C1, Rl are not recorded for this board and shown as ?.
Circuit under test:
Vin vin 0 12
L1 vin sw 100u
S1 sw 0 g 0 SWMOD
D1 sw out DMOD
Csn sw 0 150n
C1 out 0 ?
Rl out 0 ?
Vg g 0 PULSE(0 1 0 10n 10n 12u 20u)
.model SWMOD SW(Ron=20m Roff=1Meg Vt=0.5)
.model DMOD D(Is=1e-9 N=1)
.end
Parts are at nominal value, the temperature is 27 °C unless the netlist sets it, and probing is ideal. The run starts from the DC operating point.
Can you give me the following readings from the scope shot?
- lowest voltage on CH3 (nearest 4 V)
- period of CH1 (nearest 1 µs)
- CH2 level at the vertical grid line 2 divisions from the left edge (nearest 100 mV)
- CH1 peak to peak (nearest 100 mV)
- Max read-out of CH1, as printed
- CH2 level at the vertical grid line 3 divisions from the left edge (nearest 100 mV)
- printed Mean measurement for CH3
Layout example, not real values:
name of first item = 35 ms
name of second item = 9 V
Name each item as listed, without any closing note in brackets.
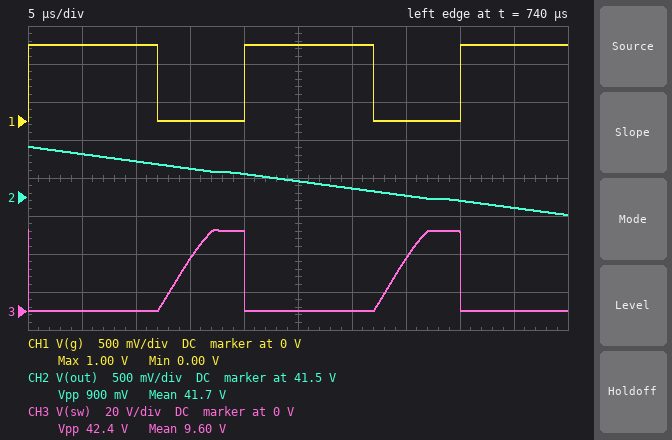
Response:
lowest voltage on CH3 = 0 V
period of CH1 = 20 µs
CH2 level at the vertical grid line 2 divisions from the left edge = 42.0 V
CH1 peak to peak = 1.0 V
Max read-out of CH1, as printed = 1.00 V
CH2 level at the vertical grid line 3 divisions from the left edge = 41.9 V
printed Mean measurement for CH3 = 9.60 V
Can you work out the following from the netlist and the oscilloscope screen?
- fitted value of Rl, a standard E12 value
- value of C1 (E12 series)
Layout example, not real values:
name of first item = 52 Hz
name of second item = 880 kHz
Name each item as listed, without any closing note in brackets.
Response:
fitted value of Rl, a standard E12 value = 56 Ω
value of C1 = 39 µF
